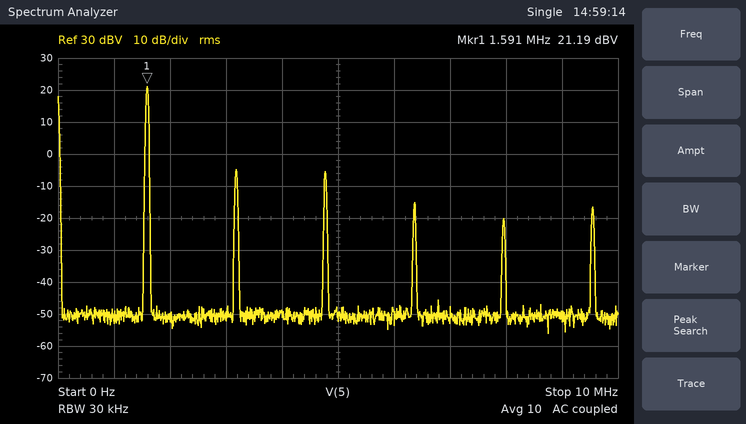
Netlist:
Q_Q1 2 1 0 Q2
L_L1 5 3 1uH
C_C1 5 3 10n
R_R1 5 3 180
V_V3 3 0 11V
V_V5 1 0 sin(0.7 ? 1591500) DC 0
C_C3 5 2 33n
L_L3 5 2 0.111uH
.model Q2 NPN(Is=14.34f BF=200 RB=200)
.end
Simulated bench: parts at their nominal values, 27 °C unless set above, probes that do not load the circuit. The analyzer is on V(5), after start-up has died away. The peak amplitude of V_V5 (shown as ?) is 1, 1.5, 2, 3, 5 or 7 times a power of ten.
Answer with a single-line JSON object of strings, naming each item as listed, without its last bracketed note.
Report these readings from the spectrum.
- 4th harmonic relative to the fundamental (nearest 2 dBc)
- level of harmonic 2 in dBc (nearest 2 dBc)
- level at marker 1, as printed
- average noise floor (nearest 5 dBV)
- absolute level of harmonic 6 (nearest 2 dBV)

{"4th harmonic relative to the fundamental": "-36 dBc", "level of harmonic 2 in dBc": "-26 dBc", "level at marker 1, as printed": "21.19 dBV", "average noise floor": "-50 dBV", "absolute level of harmonic 6": "-16 dBV"}
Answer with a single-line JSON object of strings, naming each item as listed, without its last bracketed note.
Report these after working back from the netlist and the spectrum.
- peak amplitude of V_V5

{"peak amplitude of V_V5": "1.5 V"}
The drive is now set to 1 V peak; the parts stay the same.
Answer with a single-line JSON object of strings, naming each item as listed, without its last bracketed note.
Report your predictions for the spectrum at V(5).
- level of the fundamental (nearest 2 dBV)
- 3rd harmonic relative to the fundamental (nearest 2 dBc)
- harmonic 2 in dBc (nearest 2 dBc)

{"level of the fundamental": "20 dBV", "3rd harmonic relative to the fundamental": "-28 dBc", "harmonic 2 in dBc": "-30 dBc"}
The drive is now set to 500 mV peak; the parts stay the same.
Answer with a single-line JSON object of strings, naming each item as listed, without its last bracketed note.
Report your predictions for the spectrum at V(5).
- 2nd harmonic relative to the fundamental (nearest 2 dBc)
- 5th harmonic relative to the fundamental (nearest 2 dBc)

{"2nd harmonic relative to the fundamental": "-40 dBc", "5th harmonic relative to the fundamental": "-44 dBc"}
